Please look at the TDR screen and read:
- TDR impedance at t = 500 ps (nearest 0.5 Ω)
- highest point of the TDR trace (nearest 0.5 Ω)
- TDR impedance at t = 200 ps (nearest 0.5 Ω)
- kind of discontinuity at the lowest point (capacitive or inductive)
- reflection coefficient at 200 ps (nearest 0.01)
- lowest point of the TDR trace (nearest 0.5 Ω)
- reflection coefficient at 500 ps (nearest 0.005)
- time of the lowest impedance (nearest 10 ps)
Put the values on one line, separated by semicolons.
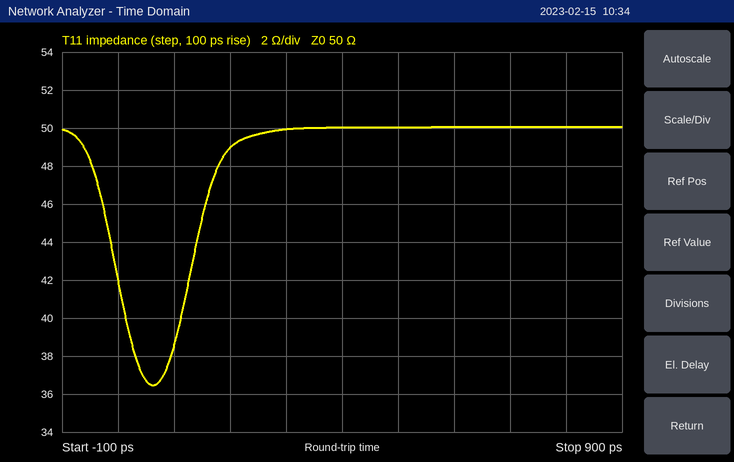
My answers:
50.0 Ω; 50.0 Ω; 49.0 Ω; capacitive; -0.01; 36.5 Ω; 0.000; 60 ps
